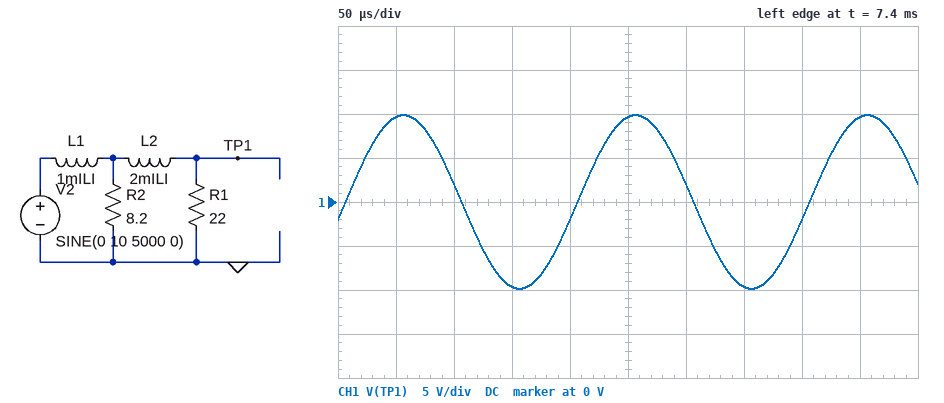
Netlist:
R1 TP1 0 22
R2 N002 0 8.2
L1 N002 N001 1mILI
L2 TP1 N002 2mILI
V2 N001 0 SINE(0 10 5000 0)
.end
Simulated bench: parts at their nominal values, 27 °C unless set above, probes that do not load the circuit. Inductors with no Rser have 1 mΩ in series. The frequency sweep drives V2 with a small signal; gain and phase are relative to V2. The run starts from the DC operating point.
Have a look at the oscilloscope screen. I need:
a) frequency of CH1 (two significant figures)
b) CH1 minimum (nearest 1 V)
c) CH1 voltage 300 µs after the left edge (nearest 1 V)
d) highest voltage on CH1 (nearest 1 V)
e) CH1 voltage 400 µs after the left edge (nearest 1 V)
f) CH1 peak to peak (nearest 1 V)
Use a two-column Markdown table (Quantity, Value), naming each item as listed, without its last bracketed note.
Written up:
| Quantity | Value |
|---|---|
| frequency of CH1 | 5.0 kHz |
| CH1 minimum | -10 V |
| CH1 voltage 300 µs after the left edge | 2 V |
| highest voltage on CH1 | 10 V |
| CH1 voltage 400 µs after the left edge | -2 V |
| CH1 peak to peak | 20 V |
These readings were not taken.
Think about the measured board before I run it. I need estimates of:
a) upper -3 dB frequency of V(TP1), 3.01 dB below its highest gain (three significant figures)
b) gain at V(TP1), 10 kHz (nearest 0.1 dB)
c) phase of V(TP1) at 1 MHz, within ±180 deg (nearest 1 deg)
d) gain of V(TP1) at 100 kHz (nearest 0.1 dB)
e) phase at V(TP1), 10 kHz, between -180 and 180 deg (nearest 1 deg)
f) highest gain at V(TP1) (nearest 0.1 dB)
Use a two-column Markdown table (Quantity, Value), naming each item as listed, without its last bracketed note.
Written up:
| Quantity | Value |
|---|---|
| upper -3 dB frequency of V(TP1), 3.01 dB below its highest gain | 28.9 kHz |
| gain at V(TP1), 10 kHz | -0.5 dB |
| phase of V(TP1) at 1 MHz, within ±180 deg | -172 deg |
| gain of V(TP1) at 100 kHz | -13.1 dB |
| phase at V(TP1), 10 kHz, between -180 and 180 deg | -23 deg |
| highest gain at V(TP1) | 0 dB |
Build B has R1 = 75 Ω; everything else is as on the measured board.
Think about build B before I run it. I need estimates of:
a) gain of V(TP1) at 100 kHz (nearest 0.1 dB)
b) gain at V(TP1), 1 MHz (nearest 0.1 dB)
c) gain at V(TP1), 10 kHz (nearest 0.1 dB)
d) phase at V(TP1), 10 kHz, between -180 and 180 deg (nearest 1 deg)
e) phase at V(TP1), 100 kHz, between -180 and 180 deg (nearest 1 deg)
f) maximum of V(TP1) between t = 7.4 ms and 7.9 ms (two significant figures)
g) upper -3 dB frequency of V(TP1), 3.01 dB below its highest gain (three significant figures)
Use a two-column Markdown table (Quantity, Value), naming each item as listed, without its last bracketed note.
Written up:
| Quantity | Value |
|---|---|
| gain of V(TP1) at 100 kHz | -8.3 dB |
| gain at V(TP1), 1 MHz | -38.7 dB |
| gain at V(TP1), 10 kHz | -0.2 dB |
| phase at V(TP1), 10 kHz, between -180 and 180 deg | -15 deg |
| phase at V(TP1), 100 kHz, between -180 and 180 deg | -86 deg |
| maximum of V(TP1) between t = 7.4 ms and 7.9 ms | 9.9 V |
| upper -3 dB frequency of V(TP1), 3.01 dB below its highest gain | 44.0 kHz |
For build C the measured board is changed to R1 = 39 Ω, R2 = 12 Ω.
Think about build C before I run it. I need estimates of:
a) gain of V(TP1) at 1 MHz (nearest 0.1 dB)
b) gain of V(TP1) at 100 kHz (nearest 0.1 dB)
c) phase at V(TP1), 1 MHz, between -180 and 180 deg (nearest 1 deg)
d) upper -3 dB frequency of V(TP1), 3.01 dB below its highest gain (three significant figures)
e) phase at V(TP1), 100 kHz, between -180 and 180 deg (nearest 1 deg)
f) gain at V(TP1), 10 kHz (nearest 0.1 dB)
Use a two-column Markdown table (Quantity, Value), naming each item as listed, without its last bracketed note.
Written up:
| Quantity | Value |
|---|---|
| gain of V(TP1) at 1 MHz | -40.9 dB |
| gain of V(TP1) at 100 kHz | -8.2 dB |
| phase at V(TP1), 1 MHz, between -180 and 180 deg | -167 deg |
| upper -3 dB frequency of V(TP1), 3.01 dB below its highest gain | 46.5 kHz |
| phase at V(TP1), 100 kHz, between -180 and 180 deg | -92 deg |
| gain at V(TP1), 10 kHz | -0.2 dB |
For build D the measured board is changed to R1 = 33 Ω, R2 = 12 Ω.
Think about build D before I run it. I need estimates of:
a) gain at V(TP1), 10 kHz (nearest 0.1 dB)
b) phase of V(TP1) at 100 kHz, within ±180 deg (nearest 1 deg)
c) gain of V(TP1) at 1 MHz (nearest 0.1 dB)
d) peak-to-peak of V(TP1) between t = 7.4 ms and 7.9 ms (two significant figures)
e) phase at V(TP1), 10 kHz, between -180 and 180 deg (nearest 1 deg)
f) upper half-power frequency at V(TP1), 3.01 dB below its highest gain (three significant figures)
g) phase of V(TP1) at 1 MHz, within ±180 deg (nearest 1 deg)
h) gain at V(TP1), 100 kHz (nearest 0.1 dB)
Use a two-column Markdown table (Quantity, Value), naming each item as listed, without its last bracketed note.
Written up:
| Quantity | Value |
|---|---|
| gain at V(TP1), 10 kHz | -0.2 dB |
| phase of V(TP1) at 100 kHz, within ±180 deg | -96 deg |
| gain of V(TP1) at 1 MHz | -42.3 dB |
| peak-to-peak of V(TP1) between t = 7.4 ms and 7.9 ms | 20 V |
| phase at V(TP1), 10 kHz, between -180 and 180 deg | -16 deg |
| upper half-power frequency at V(TP1), 3.01 dB below its highest gain | 42.8 kHz |
| phase of V(TP1) at 1 MHz, within ±180 deg | -168 deg |
| gain at V(TP1), 100 kHz | -8.9 dB |
